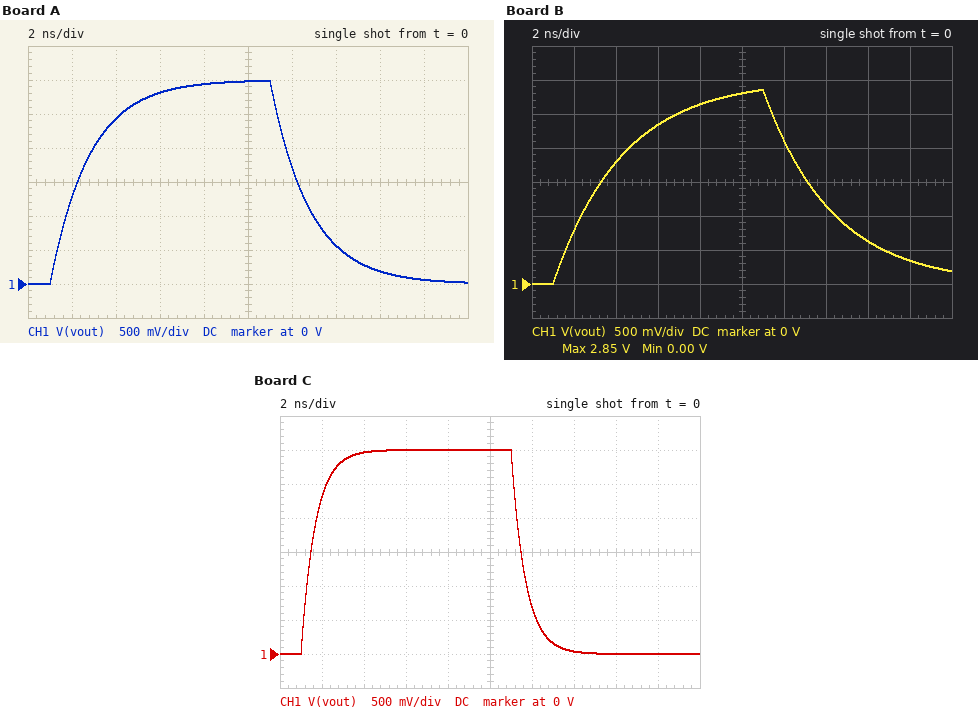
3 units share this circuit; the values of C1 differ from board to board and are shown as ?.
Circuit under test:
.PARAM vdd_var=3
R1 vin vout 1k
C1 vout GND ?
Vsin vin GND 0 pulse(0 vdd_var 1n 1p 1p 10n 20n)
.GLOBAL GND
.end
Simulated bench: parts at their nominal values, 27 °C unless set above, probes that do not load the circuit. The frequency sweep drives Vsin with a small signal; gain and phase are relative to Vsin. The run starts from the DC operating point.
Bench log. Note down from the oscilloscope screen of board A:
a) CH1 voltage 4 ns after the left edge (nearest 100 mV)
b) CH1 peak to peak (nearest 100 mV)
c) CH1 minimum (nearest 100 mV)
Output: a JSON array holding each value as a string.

["2.4 V", "3.0 V", "0 V"]
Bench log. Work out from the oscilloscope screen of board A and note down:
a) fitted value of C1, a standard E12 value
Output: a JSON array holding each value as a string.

["1.8 pF"]
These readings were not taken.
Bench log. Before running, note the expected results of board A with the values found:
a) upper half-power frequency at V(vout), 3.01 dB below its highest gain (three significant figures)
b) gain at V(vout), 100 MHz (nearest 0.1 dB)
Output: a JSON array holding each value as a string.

["88.4 MHz", "-3.6 dB"]
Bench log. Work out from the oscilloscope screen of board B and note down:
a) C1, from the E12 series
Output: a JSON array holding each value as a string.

["3.3 pF"]
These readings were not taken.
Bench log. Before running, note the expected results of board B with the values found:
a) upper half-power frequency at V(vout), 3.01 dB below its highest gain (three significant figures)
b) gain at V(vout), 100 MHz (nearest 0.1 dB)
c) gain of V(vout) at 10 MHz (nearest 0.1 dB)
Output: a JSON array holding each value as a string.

["48.2 MHz", "-7.2 dB", "-0.2 dB"]
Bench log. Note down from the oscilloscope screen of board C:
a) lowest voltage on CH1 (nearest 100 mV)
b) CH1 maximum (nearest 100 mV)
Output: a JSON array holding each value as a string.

["0 V", "3.0 V"]
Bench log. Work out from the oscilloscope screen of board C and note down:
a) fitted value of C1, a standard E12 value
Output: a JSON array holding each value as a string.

["680 fF"]
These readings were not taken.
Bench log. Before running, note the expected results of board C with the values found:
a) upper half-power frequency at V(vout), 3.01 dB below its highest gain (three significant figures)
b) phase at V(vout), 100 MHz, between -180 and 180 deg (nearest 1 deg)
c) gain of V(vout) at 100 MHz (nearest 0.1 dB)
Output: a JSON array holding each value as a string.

["234 MHz", "-23 deg", "-0.7 dB"]
